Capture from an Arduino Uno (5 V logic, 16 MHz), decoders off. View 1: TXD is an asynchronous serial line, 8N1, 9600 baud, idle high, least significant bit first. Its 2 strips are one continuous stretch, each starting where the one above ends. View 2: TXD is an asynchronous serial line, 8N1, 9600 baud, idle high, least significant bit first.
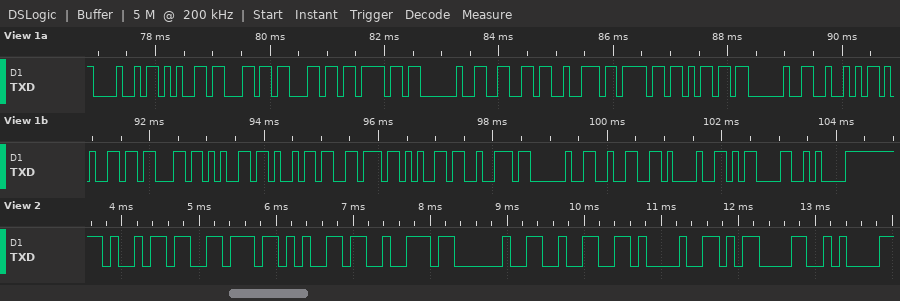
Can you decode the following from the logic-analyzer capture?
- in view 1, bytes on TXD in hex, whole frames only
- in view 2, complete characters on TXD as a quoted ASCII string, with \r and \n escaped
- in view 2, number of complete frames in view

0x48 0x65 0x6C 0x6C 0x6F 0x20 0x66 0x72 0x6F 0x6D 0x20 0x52 0x65 0x63 0x65 0x69 0x76 0x65 0x72 0x20 0x32 0x21 0x0D 0x0A
"iver 2!\r\n"
9
